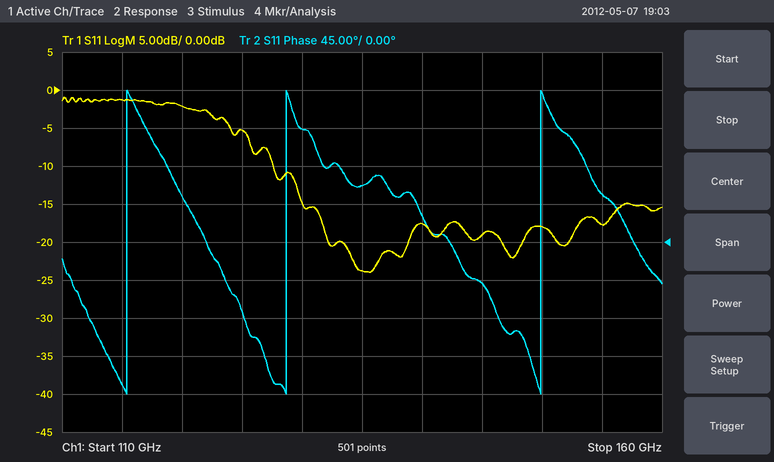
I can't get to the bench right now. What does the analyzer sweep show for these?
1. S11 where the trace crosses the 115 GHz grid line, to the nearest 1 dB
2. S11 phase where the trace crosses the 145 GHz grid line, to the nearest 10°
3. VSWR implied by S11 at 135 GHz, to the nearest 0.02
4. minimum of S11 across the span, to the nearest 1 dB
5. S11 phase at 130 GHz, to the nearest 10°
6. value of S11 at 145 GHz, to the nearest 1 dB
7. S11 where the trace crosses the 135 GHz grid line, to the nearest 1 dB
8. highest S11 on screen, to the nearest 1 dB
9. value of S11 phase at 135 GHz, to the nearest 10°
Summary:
-1 dB
-50°
1.14
-24 dB
130°
-19 dB
-24 dB
-1 dB
70°
